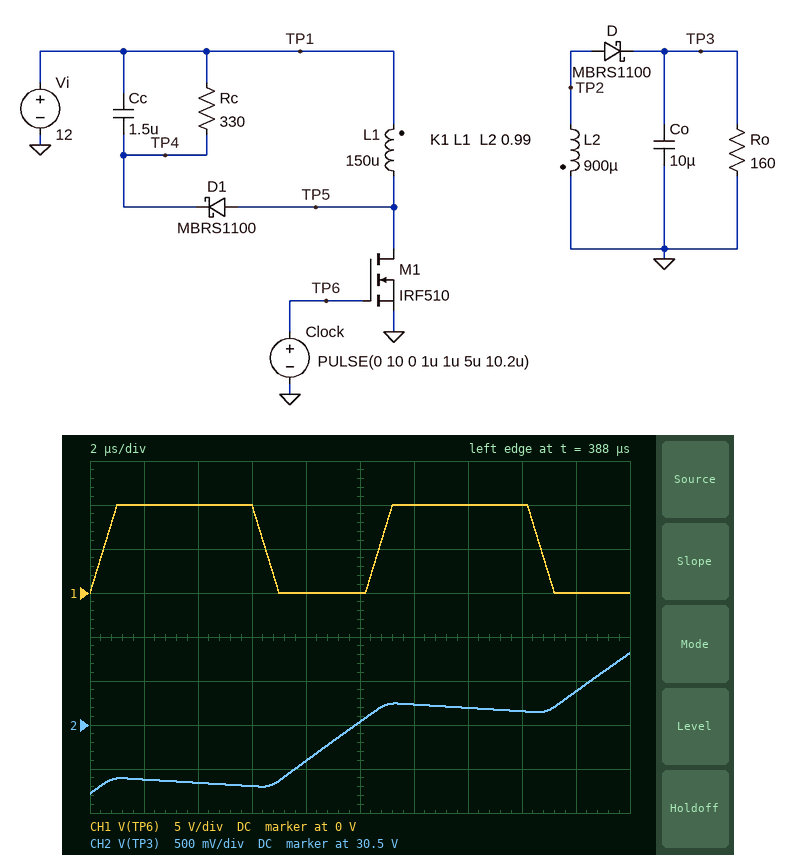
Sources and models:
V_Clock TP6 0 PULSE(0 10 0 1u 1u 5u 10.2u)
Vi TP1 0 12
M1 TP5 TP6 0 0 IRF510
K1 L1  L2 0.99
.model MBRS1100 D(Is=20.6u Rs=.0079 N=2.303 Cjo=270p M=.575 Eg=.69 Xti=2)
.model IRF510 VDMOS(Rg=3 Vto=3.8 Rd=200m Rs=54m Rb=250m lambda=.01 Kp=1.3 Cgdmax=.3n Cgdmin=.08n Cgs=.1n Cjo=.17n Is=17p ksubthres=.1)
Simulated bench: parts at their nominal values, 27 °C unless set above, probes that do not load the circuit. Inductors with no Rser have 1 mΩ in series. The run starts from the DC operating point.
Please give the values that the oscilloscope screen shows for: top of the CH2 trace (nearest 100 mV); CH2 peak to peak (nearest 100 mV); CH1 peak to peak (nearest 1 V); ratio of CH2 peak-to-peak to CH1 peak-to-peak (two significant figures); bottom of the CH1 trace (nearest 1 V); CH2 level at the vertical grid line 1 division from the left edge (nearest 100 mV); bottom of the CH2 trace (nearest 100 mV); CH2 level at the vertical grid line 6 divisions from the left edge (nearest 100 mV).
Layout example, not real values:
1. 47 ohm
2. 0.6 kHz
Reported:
1. 31.3 V
2. 1.6 V
3. 10 V
4. 0.16
5. 0 V
6. 29.9 V
7. 29.7 V
8. 30.7 V
